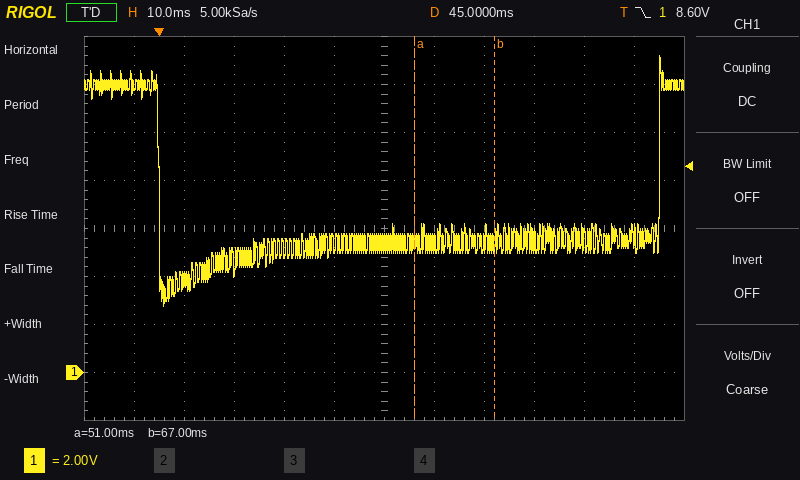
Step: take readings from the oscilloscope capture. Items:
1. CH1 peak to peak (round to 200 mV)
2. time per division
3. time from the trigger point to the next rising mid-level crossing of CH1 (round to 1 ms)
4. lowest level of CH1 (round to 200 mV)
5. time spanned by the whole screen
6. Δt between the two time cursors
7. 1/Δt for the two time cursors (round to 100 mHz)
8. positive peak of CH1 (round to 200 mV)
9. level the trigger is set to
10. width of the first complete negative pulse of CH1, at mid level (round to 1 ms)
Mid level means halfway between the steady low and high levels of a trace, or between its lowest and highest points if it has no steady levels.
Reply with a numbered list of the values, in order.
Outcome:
1. 10.4 V
2. 10 ms
3. 100 ms
4. 2.8 V
5. 120 ms
6. 16 ms
7. 62.5 Hz
8. 13.2 V
9. 8.60 V
10. 100 ms
